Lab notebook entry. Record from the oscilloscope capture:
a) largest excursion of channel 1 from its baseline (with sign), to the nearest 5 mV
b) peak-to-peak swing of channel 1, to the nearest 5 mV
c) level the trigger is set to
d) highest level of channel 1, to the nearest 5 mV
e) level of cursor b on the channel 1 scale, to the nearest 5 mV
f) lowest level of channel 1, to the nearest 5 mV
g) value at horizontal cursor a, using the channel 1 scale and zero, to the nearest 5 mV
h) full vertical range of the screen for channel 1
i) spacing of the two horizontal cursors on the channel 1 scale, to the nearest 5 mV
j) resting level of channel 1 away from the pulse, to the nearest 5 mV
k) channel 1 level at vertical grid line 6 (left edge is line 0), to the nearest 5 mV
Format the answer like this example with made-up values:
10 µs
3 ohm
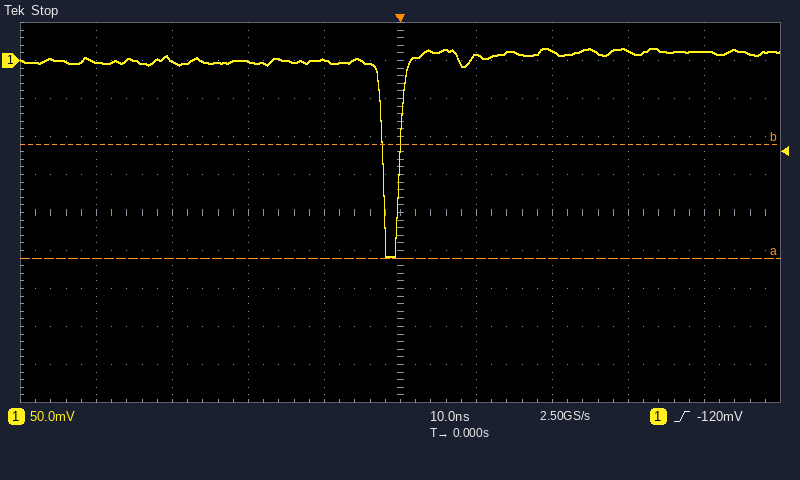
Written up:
-260 mV
275 mV
-120 mV
15 mV
-110 mV
-260 mV
-260 mV
500 mV
150 mV
0 mV
5 mV
